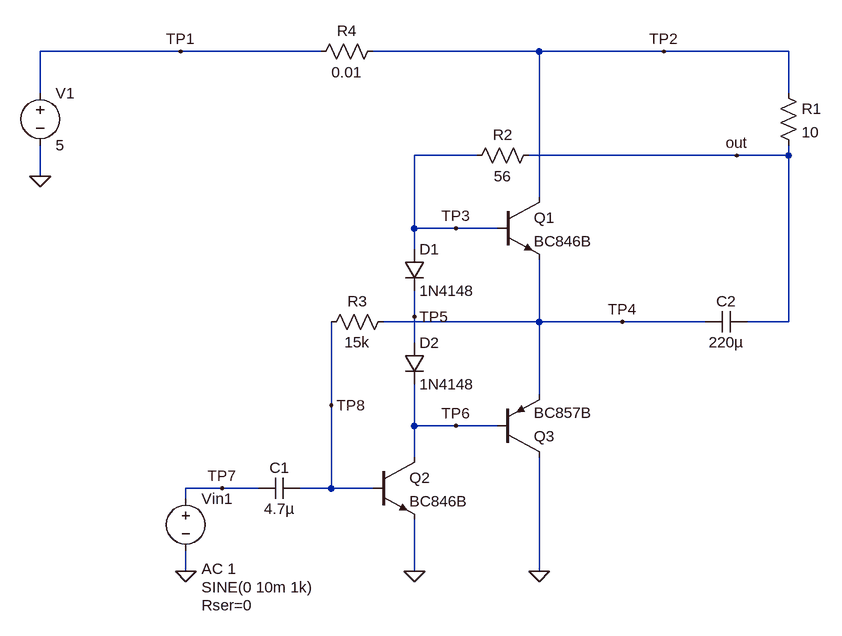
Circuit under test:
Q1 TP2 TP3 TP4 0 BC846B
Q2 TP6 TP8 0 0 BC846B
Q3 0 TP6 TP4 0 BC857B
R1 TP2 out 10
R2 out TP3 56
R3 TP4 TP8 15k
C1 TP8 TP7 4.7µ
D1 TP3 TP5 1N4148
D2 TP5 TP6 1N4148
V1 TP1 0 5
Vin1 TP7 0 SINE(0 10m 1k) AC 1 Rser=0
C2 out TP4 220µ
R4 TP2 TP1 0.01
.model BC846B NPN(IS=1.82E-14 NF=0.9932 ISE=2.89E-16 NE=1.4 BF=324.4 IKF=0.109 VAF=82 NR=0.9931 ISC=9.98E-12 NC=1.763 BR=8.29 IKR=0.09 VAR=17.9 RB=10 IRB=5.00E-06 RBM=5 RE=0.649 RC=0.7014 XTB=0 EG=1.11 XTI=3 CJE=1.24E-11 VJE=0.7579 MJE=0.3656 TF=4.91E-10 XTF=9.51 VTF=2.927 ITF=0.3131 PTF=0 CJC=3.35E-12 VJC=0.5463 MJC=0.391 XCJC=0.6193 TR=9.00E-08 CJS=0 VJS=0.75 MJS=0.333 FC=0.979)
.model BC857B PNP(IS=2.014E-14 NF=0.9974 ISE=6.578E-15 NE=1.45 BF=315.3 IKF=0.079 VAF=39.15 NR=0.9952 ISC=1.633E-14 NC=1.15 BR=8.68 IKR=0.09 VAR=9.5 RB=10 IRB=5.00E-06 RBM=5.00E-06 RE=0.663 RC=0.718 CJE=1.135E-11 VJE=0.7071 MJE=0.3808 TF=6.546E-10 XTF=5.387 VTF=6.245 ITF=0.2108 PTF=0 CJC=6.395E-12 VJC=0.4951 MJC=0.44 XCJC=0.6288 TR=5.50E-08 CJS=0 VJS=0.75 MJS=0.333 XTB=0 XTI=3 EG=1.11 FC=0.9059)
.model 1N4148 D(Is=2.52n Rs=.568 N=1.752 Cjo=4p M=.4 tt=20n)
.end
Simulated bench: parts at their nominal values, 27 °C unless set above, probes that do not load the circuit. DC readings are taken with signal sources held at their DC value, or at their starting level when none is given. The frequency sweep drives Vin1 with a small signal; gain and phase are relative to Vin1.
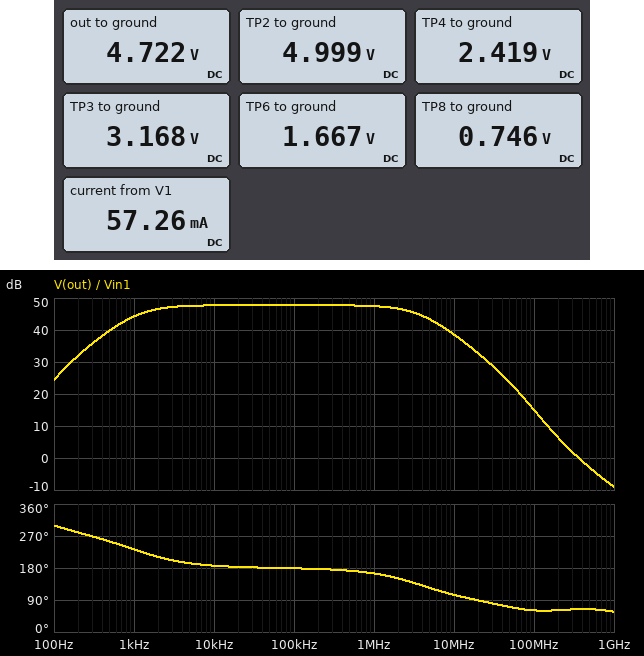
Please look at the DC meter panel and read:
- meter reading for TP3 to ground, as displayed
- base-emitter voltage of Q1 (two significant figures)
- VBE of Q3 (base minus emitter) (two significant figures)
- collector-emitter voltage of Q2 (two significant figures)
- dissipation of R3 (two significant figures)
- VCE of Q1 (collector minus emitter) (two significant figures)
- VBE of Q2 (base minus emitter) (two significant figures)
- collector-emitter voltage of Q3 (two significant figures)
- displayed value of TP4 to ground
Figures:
3.168 V
750 mV
-750 mV
1.7 V
190 µW
2.6 V
750 mV
-2.4 V
2.419 V
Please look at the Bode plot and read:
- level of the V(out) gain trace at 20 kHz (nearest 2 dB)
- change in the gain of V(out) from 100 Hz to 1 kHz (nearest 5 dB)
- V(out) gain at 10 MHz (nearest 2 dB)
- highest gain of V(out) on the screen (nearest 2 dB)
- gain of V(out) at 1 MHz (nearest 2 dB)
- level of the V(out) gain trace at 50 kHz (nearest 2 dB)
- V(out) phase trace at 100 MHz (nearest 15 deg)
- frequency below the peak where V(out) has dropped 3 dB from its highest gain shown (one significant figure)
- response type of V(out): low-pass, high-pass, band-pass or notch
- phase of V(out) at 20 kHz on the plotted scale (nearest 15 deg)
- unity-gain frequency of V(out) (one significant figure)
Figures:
48 dB
20 dB
38 dB
48 dB
48 dB
48 dB
60 deg
1 kHz
band-pass
180 deg
400 MHz
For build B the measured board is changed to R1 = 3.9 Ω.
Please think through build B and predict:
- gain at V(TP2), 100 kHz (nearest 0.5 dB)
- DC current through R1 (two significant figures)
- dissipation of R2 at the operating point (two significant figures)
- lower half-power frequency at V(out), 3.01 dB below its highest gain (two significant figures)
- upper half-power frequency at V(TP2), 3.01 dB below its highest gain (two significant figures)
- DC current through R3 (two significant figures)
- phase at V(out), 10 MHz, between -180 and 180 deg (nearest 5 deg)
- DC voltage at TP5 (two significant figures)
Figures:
-17.0 dB
29 mA
47 mW
820 Hz
3.7 MHz
120 µA
105 deg
2.5 V
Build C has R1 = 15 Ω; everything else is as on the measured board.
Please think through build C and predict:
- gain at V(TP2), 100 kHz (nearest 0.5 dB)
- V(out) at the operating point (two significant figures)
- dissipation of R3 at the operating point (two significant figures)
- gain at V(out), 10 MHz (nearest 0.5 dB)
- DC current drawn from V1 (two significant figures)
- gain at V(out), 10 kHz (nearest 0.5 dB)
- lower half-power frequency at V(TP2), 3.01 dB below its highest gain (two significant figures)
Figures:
-18.5 dB
4.6 V
170 µW
41.5 dB
55 mA
50.5 dB
1.3 kHz
